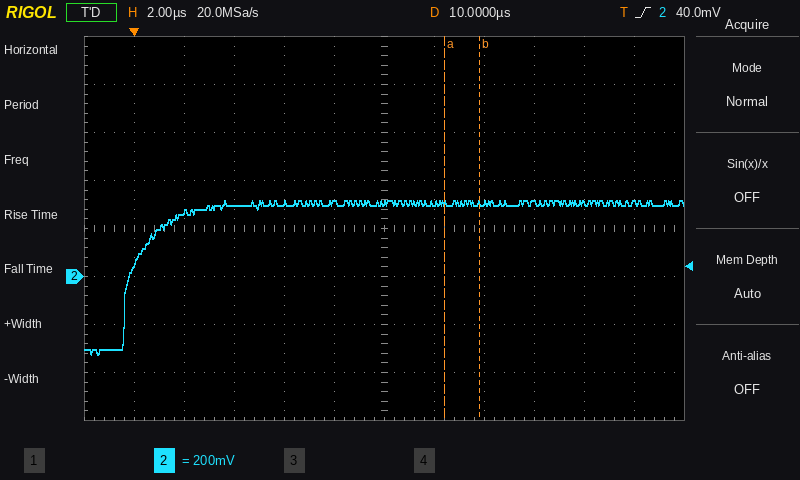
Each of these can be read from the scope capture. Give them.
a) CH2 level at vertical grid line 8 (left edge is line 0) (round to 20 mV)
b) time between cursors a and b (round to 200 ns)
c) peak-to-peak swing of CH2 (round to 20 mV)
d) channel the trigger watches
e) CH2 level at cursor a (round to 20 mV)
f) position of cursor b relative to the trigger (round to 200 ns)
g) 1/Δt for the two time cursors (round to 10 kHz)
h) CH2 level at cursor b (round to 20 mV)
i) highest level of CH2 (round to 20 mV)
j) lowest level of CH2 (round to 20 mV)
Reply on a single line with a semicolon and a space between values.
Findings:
300 mV; 1.4 µs; 640 mV; CH2; 300 mV; +13.8 µs; 710 kHz; 300 mV; 320 mV; -320 mV
